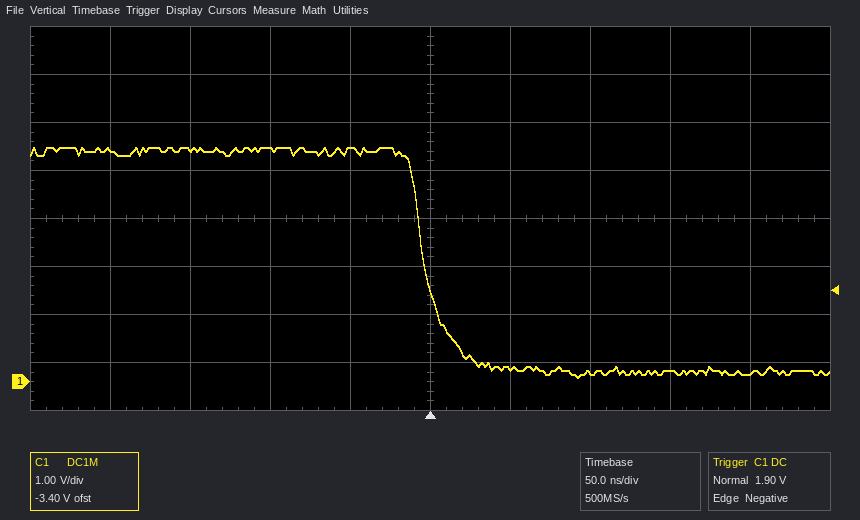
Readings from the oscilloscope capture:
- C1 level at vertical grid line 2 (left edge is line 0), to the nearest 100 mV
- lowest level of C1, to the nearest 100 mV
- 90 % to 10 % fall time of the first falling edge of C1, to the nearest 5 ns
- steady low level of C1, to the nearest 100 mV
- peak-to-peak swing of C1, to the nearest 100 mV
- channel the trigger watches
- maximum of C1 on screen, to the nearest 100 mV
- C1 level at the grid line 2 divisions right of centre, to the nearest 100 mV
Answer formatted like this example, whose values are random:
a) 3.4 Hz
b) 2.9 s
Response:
a) 4.8 V
b) 100 mV
c) 30 ns
d) 200 mV
e) 4.8 V
f) C1
g) 4.9 V
h) 200 mV
